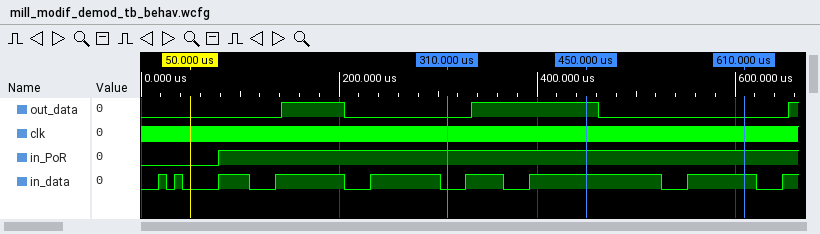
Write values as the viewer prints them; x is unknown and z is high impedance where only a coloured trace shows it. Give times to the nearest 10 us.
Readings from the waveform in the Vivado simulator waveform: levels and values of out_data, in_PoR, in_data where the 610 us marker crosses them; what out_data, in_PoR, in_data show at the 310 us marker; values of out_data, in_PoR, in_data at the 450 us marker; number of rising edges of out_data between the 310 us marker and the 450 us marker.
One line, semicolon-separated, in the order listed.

out_data=0, in_PoR=1, in_data=1; out_data=0, in_PoR=1, in_data=0; out_data=1, in_PoR=1, in_data=1; 1
